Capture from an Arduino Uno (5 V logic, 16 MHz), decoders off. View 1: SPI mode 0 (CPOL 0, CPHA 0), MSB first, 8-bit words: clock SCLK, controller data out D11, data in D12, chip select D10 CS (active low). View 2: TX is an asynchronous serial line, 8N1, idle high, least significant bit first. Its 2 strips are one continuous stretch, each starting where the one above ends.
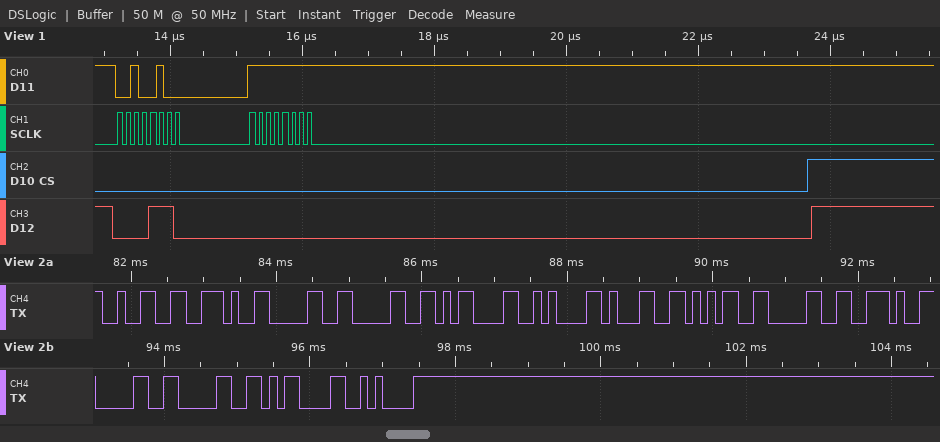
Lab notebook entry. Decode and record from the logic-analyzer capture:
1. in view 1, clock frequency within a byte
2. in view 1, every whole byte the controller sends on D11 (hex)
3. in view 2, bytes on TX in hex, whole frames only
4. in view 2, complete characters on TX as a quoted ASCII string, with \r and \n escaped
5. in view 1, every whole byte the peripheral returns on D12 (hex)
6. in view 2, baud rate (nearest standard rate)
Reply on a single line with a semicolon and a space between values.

8 MHz; 24 FF; 32 2E 30 30 0D 0A 31 35 30 2E 30 30 0D 0A; "2.00\r\n150.00\r\n"; 0E 00; 9600 baud
